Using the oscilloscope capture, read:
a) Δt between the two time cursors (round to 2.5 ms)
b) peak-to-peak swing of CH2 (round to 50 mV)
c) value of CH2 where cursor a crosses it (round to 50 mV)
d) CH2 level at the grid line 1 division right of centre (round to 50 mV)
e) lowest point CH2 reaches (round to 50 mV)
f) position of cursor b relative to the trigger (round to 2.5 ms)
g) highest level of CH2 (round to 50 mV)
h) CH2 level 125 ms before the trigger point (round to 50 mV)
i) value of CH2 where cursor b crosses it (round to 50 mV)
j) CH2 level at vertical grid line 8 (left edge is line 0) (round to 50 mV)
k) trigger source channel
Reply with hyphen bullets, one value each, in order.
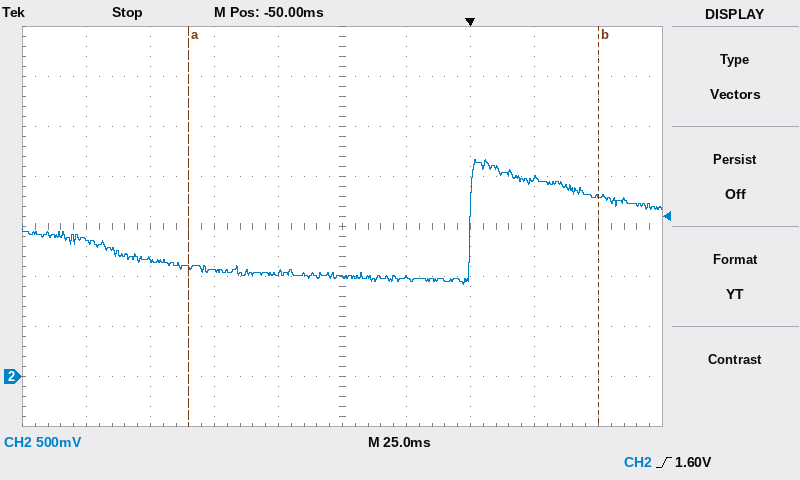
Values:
- 160.0 ms
- 1.25 V
- 1.10 V
- 1.00 V
- 900 mV
- +50.0 ms
- 2.15 V
- 1.15 V
- 1.80 V
- 2.00 V
- CH2
